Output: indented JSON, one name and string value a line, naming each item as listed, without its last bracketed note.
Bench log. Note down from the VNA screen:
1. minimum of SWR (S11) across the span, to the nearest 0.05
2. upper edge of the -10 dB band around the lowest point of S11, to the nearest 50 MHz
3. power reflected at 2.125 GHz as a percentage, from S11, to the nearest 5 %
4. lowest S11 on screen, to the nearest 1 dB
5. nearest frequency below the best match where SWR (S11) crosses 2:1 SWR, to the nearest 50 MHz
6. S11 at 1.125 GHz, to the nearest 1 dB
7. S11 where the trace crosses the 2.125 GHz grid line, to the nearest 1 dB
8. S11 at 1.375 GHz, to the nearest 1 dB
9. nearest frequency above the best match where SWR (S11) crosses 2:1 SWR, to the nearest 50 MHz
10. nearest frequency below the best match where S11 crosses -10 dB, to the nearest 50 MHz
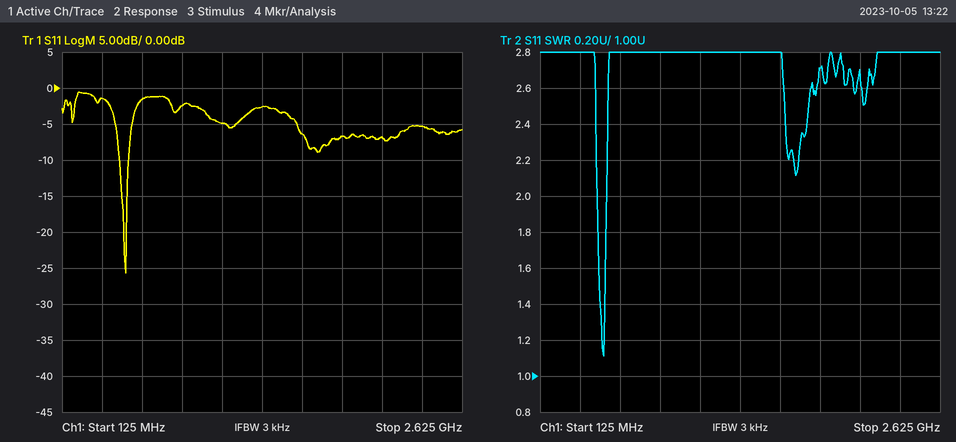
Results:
{
  "minimum of SWR (S11) across the span, to the nearest 0.05": "1.10",
  "upper edge of the -10 dB band around the lowest point of S11, to the nearest 50 MHz": "550 MHz",
  "power reflected at 2.125 GHz as a percentage, from S11, to the nearest 5 %": "20 %",
  "lowest S11 on screen, to the nearest 1 dB": "-26 dB",
  "nearest frequency below the best match where SWR (S11) crosses 2:1 SWR, to the nearest 50 MHz": "500 MHz",
  "S11 at 1.125 GHz, to the nearest 1 dB": "-5 dB",
  "S11 where the trace crosses the 2.125 GHz grid line, to the nearest 1 dB": "-7 dB",
  "S11 at 1.375 GHz, to the nearest 1 dB": "-3 dB",
  "nearest frequency above the best match where SWR (S11) crosses 2:1 SWR, to the nearest 50 MHz": "550 MHz",
  "nearest frequency below the best match where S11 crosses -10 dB, to the nearest 50 MHz": "500 MHz"
}
